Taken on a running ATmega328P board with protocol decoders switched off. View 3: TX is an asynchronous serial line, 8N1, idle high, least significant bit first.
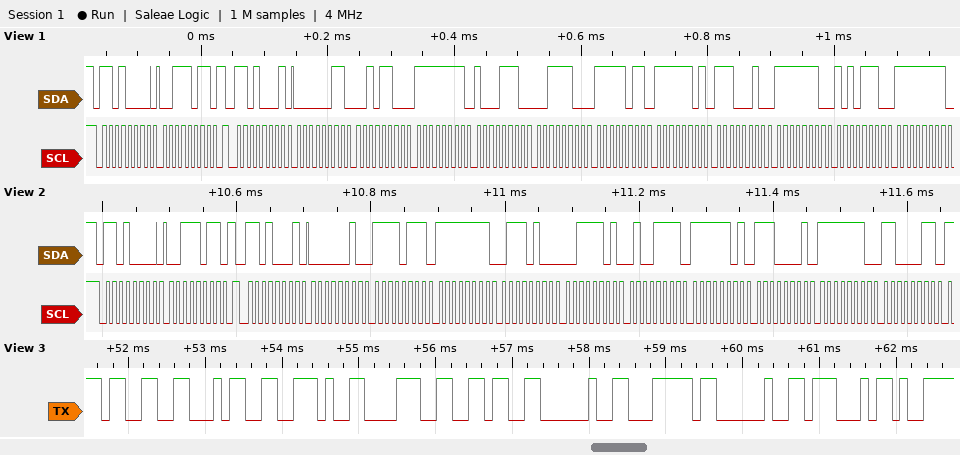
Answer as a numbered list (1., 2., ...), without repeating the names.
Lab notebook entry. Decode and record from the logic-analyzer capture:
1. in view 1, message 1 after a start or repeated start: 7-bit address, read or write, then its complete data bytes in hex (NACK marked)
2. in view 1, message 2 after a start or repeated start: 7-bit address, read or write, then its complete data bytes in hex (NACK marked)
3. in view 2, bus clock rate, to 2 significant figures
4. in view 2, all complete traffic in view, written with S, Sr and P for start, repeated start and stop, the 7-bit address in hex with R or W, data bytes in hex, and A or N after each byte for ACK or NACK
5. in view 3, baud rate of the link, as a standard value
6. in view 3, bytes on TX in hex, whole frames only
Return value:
1. 0x68 write: 3B
2. 0x68 read: 03 2C FF 8E 3C FB FD E2 FE AE FF
3. 100 kHz
4. S 68W A 3B A Sr 68R A 02 A F7 A FF A 74 A 3D A 4F A FD A E1 A FE A C3 A
5. 9600 baud
6. 33 34 2E 38 36 20 7C 20 47
